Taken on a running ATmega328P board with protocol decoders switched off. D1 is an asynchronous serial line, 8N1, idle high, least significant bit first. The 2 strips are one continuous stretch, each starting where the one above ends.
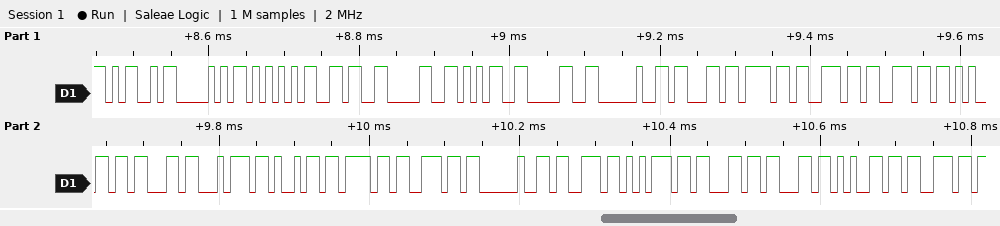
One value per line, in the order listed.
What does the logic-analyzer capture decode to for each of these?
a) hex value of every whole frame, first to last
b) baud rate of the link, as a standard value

4D 50 55 36 30 35 30 20 63 6F 6E 6E 65 63 74 69 6F 6E 20 73 75 63 63 65 73
115200 baud
